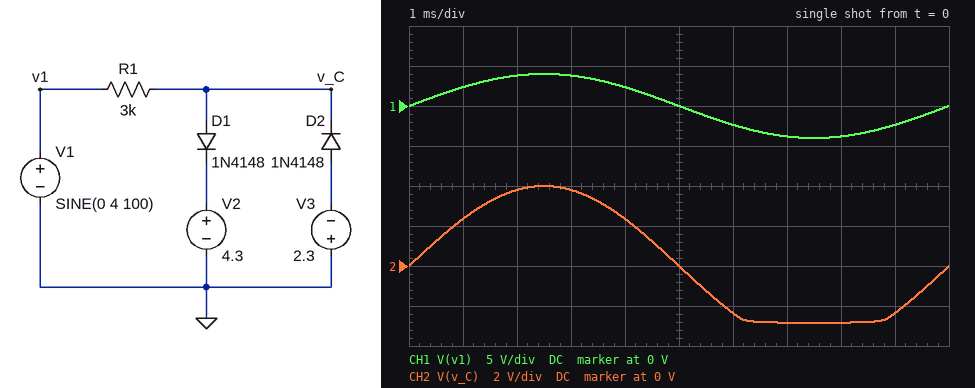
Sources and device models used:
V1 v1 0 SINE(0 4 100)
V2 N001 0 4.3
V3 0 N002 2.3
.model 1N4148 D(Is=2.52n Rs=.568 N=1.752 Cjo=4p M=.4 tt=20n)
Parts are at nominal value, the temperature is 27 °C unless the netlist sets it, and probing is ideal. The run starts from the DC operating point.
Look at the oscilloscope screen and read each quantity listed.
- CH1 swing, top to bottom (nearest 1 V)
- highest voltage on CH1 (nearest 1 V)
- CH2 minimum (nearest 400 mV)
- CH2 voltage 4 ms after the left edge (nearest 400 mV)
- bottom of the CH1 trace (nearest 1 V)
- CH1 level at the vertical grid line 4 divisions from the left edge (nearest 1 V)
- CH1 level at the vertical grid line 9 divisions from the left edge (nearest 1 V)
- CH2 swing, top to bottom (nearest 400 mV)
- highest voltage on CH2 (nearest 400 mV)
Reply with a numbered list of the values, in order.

1. 8 V
2. 4 V
3. -2.8 V
4. 2.4 V
5. -4 V
6. 2 V
7. -2 V
8. 6.8 V
9. 4.0 V
